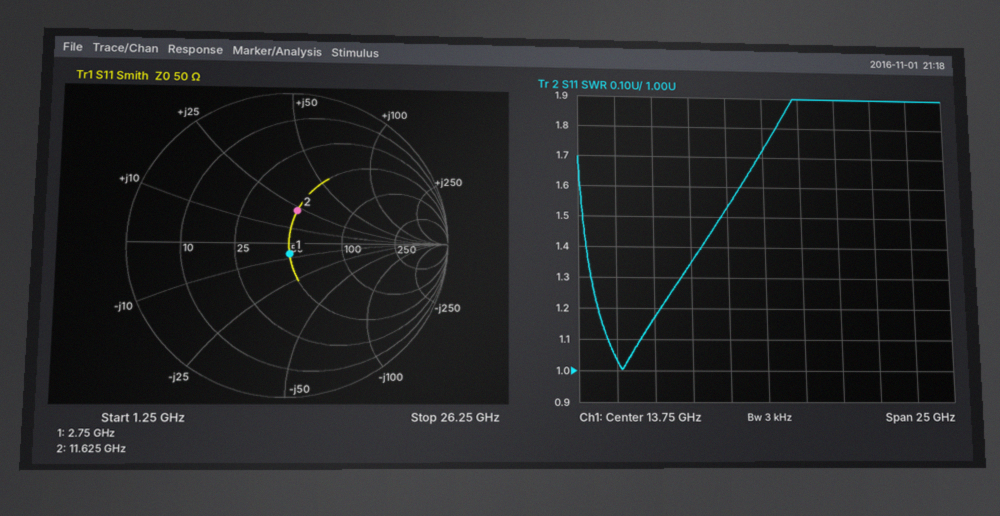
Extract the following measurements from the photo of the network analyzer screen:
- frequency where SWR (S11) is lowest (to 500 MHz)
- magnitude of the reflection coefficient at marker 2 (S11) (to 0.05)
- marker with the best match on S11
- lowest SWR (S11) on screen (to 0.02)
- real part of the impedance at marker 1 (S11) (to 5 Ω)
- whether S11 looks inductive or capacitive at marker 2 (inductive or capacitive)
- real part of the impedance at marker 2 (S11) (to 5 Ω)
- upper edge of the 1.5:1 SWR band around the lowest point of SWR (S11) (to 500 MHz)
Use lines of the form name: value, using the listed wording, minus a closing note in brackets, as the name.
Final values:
frequency where SWR (S11) is lowest: 4.0 GHz
magnitude of the reflection coefficient at marker 2 (S11): 0.20
marker with the best match on S11: marker 1
lowest SWR (S11) on screen: 1.00
real part of the impedance at marker 1 (S11): 50 Ω
whether S11 looks inductive or capacitive at marker 2: inductive
real part of the impedance at marker 2 (S11): 50 Ω
upper edge of the 1.5:1 SWR band around the lowest point of SWR (S11): 11.0 GHz
